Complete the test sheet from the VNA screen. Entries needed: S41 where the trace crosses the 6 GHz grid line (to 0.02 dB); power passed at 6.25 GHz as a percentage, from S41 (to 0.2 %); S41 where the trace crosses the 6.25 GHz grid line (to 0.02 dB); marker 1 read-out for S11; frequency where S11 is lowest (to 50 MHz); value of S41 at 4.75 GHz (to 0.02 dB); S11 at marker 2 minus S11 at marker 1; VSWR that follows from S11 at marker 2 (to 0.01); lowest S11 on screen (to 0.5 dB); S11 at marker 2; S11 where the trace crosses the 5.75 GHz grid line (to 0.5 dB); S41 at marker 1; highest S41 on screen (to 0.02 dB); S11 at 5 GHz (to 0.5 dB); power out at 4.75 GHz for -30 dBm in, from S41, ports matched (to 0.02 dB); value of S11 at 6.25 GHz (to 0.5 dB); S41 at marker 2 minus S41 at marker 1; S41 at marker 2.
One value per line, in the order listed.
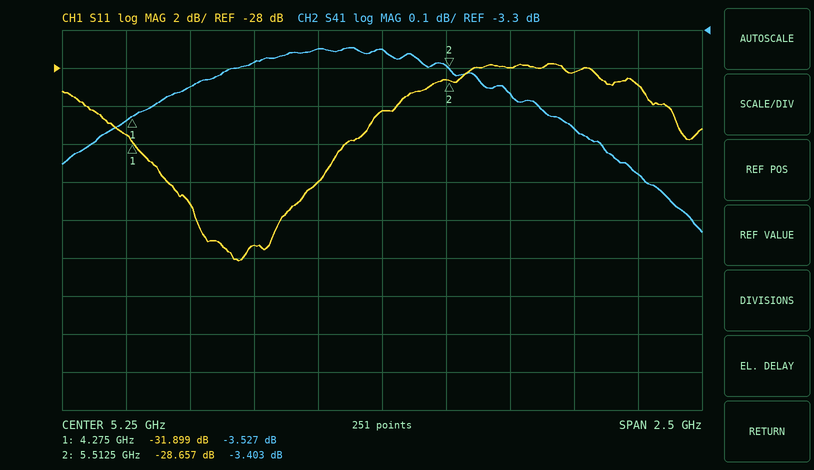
-3.56 dB
42.8 %
-3.68 dB
-31.899 dB
4.70 GHz
-3.38 dB
3.242 dB
1.08
-38.0 dB
-28.657 dB
-28.0 dB
-3.527 dB
-3.34 dB
-34.0 dB
-33.38 dBm
-29.0 dB
0.124 dB
-3.403 dB
